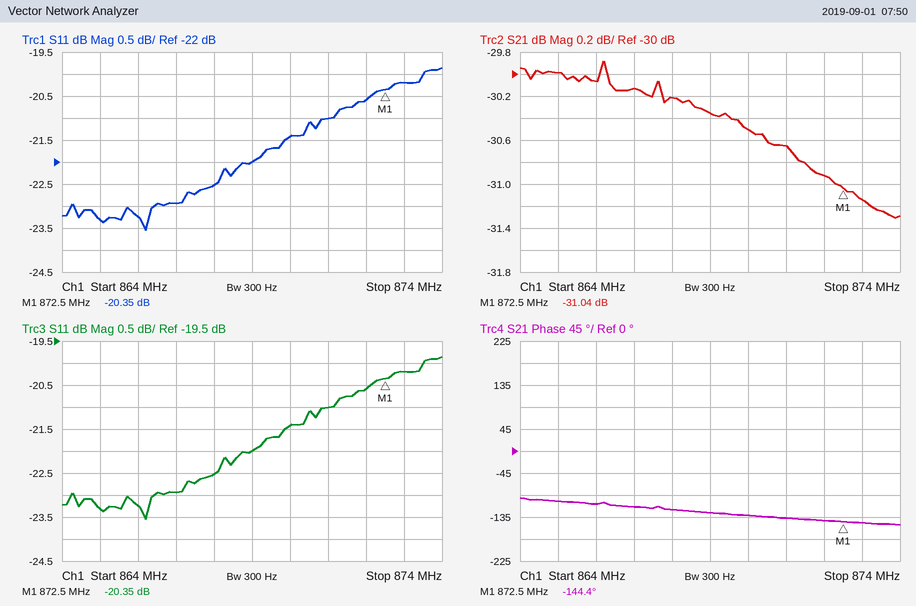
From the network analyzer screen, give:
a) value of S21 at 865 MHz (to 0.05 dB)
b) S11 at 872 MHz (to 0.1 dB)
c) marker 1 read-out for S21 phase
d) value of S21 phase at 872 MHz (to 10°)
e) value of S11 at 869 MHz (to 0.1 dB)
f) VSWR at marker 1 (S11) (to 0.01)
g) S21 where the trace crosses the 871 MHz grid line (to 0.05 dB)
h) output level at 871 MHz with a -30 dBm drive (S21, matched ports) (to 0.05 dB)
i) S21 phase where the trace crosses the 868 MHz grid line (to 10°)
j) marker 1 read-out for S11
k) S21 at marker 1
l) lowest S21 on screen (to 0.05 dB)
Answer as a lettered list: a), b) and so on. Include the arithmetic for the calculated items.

a) -30.00 dB
b) -20.6 dB
c) -144.4°
d) -140°
e) -22.0 dB
f) (1 + 0.0961)/(1 − 0.0961) ≈ 1.21
g) -30.65 dB
h) -30 dBm + (-30.65 dB) = -60.65 dBm
i) -120°
j) -20.35 dB
k) -31.04 dB
l) -31.30 dB
